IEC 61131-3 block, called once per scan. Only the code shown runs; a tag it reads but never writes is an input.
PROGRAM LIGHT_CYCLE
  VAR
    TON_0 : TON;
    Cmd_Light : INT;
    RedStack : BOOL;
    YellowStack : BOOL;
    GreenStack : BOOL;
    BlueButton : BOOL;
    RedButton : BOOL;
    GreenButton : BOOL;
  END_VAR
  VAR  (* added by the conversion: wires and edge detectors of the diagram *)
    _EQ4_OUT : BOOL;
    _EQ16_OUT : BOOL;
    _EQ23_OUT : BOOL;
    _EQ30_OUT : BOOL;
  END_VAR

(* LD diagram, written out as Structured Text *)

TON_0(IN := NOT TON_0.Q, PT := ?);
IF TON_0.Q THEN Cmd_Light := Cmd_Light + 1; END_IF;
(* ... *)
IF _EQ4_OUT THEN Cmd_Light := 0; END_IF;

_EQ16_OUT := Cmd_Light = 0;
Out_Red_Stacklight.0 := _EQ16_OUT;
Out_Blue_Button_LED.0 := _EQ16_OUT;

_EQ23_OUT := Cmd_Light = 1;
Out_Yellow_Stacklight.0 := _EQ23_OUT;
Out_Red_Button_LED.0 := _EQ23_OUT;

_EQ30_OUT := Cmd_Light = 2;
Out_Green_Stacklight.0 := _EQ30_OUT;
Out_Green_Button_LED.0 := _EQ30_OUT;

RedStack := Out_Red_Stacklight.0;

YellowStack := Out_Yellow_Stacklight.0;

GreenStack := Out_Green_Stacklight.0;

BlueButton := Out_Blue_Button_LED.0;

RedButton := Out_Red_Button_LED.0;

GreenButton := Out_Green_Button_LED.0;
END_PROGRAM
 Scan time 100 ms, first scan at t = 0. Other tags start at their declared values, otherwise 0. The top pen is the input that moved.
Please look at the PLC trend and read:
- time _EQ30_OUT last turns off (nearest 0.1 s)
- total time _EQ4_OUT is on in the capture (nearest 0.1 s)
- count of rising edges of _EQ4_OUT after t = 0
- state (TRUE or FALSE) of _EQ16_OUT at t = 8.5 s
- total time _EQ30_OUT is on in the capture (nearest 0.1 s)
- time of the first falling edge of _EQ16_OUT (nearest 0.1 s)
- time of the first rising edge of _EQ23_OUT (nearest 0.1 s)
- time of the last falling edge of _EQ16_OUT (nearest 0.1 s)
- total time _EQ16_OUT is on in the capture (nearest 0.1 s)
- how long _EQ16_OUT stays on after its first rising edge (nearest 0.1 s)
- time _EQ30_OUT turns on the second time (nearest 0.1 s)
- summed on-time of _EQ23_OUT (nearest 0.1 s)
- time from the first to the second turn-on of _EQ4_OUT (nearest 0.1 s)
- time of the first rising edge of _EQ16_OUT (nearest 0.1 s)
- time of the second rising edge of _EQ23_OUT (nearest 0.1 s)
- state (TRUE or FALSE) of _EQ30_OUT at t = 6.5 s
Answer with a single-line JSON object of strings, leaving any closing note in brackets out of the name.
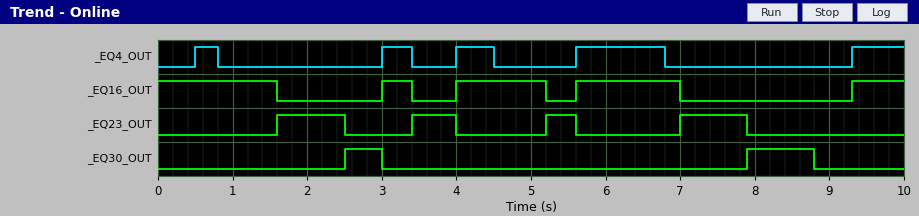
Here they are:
{"time _EQ30_OUT last turns off": "8.8 s", "total time _EQ4_OUT is on in the capture": "3.1 s", "count of rising edges of _EQ4_OUT after t = 0": "5", "state (TRUE or FALSE) of _EQ16_OUT at t = 8.5 s": "FALSE", "total time _EQ30_OUT is on in the capture": "1.4 s", "time of the first falling edge of _EQ16_OUT": "1.6 s", "time of the first rising edge of _EQ23_OUT": "1.6 s", "time of the last falling edge of _EQ16_OUT": "7.0 s", "total time _EQ16_OUT is on in the capture": "5.3 s", "how long _EQ16_OUT stays on after its first rising edge": "0.4 s", "time _EQ30_OUT turns on the second time": "7.9 s", "summed on-time of _EQ23_OUT": "2.8 s", "time from the first to the second turn-on of _EQ4_OUT": "2.5 s", "time of the first rising edge of _EQ16_OUT": "3.0 s", "time of the second rising edge of _EQ23_OUT": "3.4 s", "state (TRUE or FALSE) of _EQ30_OUT at t = 6.5 s": "FALSE"}
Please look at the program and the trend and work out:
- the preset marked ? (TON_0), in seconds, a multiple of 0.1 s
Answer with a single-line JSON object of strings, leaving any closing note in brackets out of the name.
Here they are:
{"the preset marked ? (TON_0), in seconds, a multiple of 0.1 s": "0.7 s"}
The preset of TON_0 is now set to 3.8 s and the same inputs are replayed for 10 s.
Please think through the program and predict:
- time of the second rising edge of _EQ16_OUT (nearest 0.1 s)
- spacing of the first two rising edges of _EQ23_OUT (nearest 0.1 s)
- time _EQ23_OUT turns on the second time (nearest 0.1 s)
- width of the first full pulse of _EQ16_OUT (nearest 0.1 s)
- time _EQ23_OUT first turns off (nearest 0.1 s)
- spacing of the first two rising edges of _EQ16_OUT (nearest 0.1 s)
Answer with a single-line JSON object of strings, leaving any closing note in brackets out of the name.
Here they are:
{"time of the second rising edge of _EQ16_OUT": "9.3 s", "spacing of the first two rising edges of _EQ23_OUT": "4.0 s", "time _EQ23_OUT turns on the second time": "7.8 s", "width of the first full pulse of _EQ16_OUT": "3.8 s", "time _EQ23_OUT first turns off": "4.0 s", "spacing of the first two rising edges of _EQ16_OUT": "5.3 s"}
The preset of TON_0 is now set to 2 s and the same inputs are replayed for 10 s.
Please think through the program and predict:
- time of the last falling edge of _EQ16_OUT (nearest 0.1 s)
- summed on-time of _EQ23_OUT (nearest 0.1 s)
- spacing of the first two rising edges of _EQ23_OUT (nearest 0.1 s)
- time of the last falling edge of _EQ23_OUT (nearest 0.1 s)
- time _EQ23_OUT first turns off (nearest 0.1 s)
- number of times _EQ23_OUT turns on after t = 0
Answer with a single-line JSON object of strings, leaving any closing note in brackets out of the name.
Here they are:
{"time of the last falling edge of _EQ16_OUT": "8.6 s", "summed on-time of _EQ23_OUT": "1.7 s", "spacing of the first two rising edges of _EQ23_OUT": "6.6 s", "time of the last falling edge of _EQ23_OUT": "9.3 s", "time _EQ23_OUT first turns off": "3.0 s", "number of times _EQ23_OUT turns on after t = 0": "2"}
